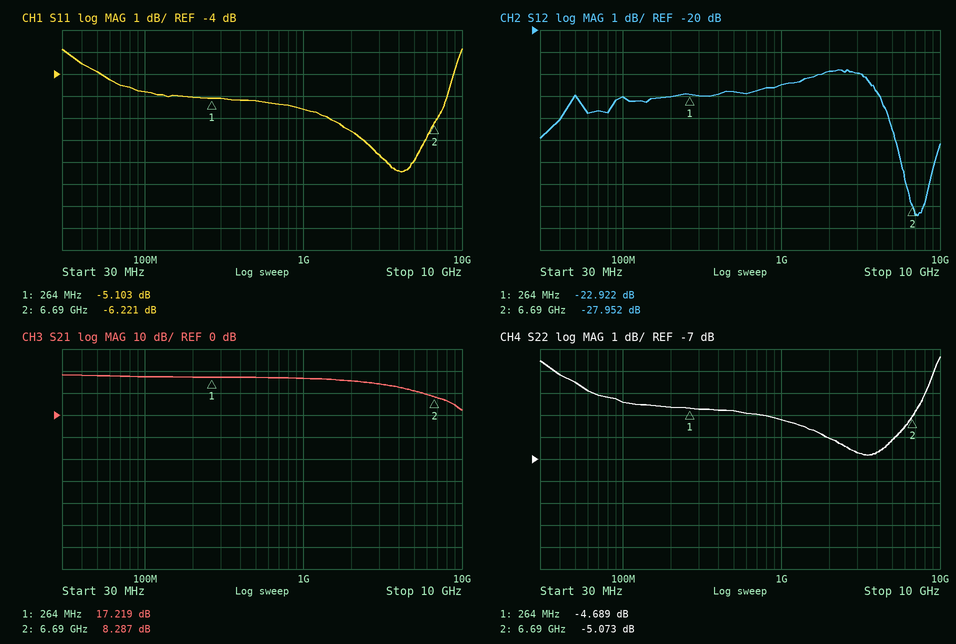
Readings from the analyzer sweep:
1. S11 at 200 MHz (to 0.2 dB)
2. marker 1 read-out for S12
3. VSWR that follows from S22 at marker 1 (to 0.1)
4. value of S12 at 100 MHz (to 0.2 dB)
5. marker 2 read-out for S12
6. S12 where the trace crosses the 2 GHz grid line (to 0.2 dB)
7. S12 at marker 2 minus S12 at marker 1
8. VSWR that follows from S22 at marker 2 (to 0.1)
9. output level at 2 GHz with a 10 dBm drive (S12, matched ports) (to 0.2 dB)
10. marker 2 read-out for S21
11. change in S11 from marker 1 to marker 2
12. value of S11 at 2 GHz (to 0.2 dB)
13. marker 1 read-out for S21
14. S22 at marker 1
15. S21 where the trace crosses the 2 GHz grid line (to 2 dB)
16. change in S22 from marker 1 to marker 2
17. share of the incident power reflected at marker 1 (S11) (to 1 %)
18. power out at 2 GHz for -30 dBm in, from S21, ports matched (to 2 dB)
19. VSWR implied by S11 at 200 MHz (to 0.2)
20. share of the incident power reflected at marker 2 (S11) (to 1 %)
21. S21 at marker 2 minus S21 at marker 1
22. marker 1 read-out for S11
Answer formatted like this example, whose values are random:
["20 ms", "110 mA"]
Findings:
["-5.0 dB", "-22.922 dB", "3.8", "-23.0 dB", "-27.952 dB", "-21.8 dB", "-5.030 dB", "3.5", "-11.8 dBm", "8.287 dB", "-1.118 dB", "-6.6 dB", "17.219 dB", "-4.689 dB", "16 dB", "-0.384 dB", "31 %", "-14 dBm", "3.6", "24 %", "-8.932 dB", "-5.103 dB"]
